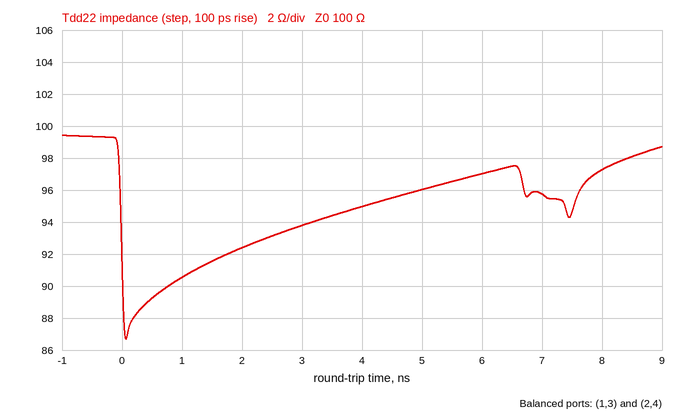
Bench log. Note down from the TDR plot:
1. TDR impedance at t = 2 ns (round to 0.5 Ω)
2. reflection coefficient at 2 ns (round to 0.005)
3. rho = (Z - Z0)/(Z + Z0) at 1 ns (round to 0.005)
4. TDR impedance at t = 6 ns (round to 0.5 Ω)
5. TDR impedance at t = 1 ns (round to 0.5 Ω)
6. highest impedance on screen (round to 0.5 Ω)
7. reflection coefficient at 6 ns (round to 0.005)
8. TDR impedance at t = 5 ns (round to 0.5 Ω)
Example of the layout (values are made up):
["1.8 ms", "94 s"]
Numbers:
["92.5 Ω", "-0.040", "-0.050", "97.0 Ω", "90.5 Ω", "99.5 Ω", "-0.015", "96.0 Ω"]
